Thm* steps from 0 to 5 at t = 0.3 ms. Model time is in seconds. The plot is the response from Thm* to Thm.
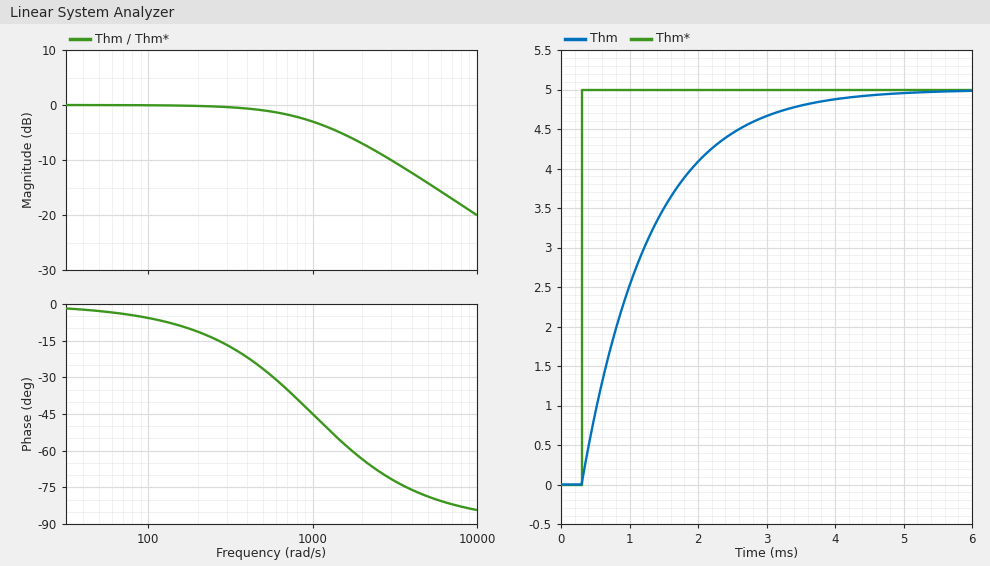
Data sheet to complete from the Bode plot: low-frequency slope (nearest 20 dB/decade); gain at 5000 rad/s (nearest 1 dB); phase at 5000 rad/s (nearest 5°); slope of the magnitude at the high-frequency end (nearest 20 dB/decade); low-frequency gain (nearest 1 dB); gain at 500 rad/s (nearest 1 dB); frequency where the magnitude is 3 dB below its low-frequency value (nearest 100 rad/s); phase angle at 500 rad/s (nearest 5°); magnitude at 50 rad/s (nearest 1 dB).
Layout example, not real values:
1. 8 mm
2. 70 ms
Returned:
1. 0 dB/decade
2. -14 dB
3. -80°
4. -20 dB/decade
5. 0 dB
6. -1 dB
7. 1000 rad/s
8. -25°
9. 0 dB
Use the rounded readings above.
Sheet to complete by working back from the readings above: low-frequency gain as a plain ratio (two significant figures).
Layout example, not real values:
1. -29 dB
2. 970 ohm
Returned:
1. 1.0
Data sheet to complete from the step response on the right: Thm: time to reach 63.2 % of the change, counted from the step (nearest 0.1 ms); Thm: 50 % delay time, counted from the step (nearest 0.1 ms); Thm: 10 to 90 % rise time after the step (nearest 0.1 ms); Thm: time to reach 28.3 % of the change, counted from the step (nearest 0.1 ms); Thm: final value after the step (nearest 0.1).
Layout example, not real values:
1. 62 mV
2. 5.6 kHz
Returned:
1. 1.0 ms
2. 0.7 ms
3. 2.2 ms
4. 0.3 ms
5. 5.0
